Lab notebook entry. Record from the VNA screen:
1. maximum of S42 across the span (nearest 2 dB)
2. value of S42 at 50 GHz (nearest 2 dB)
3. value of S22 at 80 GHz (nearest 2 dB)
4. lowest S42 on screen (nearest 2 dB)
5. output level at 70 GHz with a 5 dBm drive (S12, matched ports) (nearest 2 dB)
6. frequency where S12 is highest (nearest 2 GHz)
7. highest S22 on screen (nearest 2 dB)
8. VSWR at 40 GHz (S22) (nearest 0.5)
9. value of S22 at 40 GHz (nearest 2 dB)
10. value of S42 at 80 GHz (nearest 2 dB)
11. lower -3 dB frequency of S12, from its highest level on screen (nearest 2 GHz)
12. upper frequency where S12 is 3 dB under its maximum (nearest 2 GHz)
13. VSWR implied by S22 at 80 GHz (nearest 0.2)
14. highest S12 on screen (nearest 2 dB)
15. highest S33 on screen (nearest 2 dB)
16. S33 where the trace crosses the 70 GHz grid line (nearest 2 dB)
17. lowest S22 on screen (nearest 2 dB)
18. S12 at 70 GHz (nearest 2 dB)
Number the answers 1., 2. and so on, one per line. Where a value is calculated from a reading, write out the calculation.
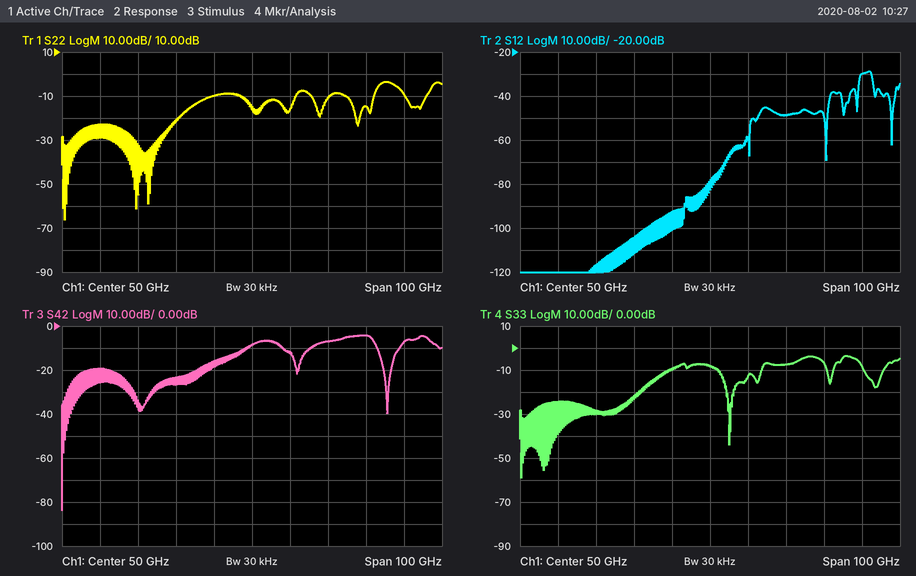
1. -4 dB
2. -8 dB
3. -14 dB
4. -84 dB
5. 5 dBm + (-48 dB) = -44 dBm
6. 92 GHz
7. -4 dB
8. |Γ| = 10^(-10/20) = 0.3162; VSWR = (1 + 0.3162)/(1 − 0.3162) ≈ 1.92, so 2.0 to the nearest 0.5
9. -10 dB
10. -4 dB
11. 90 GHz
12. 92 GHz
13. |Γ| = 10^(-14/20) = 0.1995; VSWR = (1 + 0.1995)/(1 − 0.1995) ≈ 1.50, so 1.4 to the nearest 0.2
14. -28 dB
15. -4 dB
16. -8 dB
17. -66 dB
18. -48 dB
